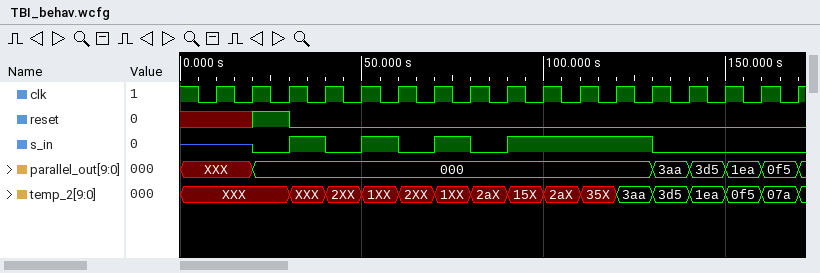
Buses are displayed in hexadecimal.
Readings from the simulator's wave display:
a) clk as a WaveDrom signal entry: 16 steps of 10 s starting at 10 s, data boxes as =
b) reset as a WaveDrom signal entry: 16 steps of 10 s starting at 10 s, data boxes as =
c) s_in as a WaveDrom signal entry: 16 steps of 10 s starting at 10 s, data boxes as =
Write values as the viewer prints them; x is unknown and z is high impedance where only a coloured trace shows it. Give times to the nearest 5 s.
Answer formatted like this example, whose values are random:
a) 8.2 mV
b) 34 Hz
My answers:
a) {name: 'clk', wave: 'p...............'}
b) {name: 'reset', wave: 'x10.............'}
c) {name: 's_in', wave: 'z01010101...0...'}
